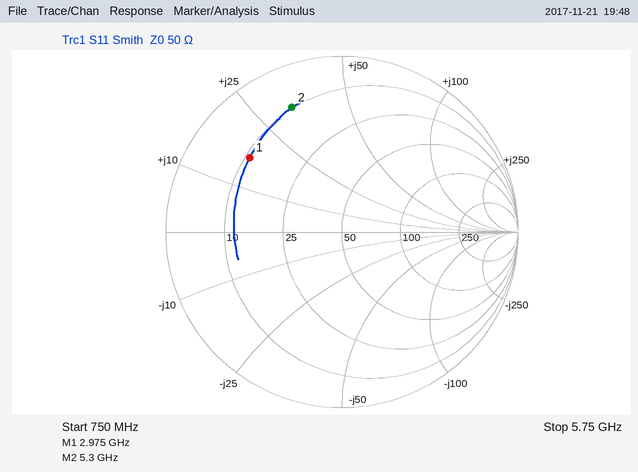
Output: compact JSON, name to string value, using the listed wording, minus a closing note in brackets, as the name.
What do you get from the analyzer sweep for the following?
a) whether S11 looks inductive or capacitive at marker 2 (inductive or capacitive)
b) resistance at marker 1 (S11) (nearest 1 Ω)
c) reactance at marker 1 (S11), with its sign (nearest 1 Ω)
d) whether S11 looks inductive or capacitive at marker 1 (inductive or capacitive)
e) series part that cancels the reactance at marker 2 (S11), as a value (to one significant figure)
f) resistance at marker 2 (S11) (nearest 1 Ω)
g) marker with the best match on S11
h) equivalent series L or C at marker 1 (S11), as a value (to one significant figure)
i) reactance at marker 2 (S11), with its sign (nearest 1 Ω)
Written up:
{"whether S11 looks inductive or capacitive at marker 2": "inductive", "resistance at marker 1 (S11)": "11 Ω", "reactance at marker 1 (S11), with its sign": "+17 Ω", "whether S11 looks inductive or capacitive at marker 1": "inductive", "series part that cancels the reactance at marker 2 (S11), as a value": "900 fF", "resistance at marker 2 (S11)": "10 Ω", "marker with the best match on S11": "marker 1", "equivalent series L or C at marker 1 (S11), as a value": "900 pH", "reactance at marker 2 (S11), with its sign": "+33 Ω"}
